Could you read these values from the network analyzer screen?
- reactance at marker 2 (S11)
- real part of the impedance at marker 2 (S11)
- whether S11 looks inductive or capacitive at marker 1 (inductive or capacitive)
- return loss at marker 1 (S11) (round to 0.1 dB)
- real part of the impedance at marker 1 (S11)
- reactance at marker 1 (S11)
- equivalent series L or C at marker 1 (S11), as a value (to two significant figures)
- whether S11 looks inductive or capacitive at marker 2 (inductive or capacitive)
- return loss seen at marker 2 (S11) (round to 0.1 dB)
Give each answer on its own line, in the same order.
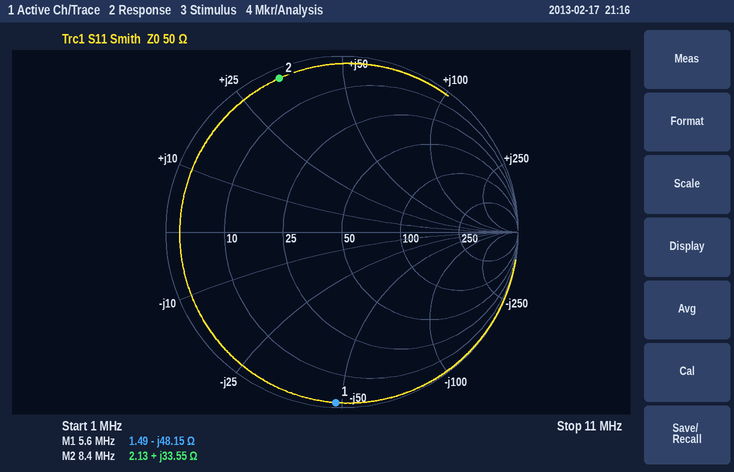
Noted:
+33.55 Ω
2.13 Ω
capacitive
0.3 dB
1.49 Ω
-48.15 Ω
590 pF
inductive
0.5 dB
